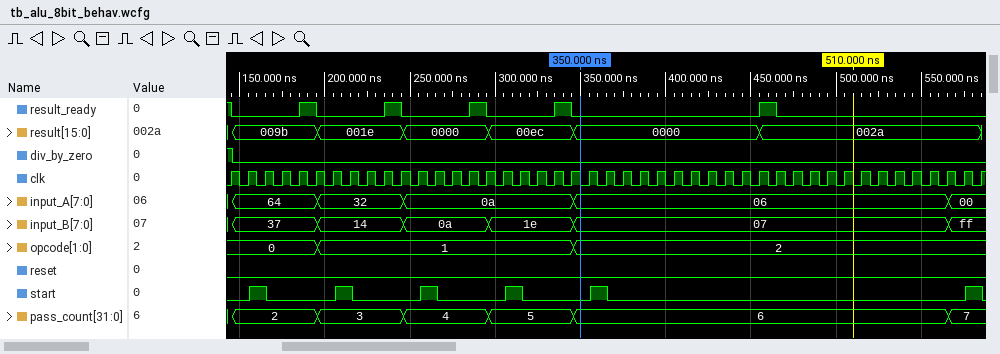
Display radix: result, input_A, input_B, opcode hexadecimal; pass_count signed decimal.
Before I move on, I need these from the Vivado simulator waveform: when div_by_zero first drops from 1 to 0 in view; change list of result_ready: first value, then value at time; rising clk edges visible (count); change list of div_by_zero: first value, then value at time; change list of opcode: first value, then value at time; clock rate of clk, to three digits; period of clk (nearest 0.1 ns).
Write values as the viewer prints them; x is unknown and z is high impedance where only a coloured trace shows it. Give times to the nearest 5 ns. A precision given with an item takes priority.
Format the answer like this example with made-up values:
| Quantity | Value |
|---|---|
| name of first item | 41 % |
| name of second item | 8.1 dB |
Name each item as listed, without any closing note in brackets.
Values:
| Quantity | Value |
|---|---|
| when div_by_zero first drops from 1 to 0 in view | 145 ns |
| change list of result_ready: first value, then value at time | 1, 0 at 145 ns, 1 at 185 ns, 0 at 195 ns, 1 at 235 ns, 0 at 245 ns, 1 at 285 ns, 0 at 295 ns, 1 at 335 ns, 0 at 345 ns, 1 at 455 ns, 0 at 465 ns |
| rising clk edges visible | 45 |
| change list of div_by_zero: first value, then value at time | 1, 0 at 145 ns |
| change list of opcode: first value, then value at time | 0, 1 at 195 ns, 2 at 345 ns |
| clock rate of clk, to three digits | 100 MHz |
| period of clk | 10 ns |
